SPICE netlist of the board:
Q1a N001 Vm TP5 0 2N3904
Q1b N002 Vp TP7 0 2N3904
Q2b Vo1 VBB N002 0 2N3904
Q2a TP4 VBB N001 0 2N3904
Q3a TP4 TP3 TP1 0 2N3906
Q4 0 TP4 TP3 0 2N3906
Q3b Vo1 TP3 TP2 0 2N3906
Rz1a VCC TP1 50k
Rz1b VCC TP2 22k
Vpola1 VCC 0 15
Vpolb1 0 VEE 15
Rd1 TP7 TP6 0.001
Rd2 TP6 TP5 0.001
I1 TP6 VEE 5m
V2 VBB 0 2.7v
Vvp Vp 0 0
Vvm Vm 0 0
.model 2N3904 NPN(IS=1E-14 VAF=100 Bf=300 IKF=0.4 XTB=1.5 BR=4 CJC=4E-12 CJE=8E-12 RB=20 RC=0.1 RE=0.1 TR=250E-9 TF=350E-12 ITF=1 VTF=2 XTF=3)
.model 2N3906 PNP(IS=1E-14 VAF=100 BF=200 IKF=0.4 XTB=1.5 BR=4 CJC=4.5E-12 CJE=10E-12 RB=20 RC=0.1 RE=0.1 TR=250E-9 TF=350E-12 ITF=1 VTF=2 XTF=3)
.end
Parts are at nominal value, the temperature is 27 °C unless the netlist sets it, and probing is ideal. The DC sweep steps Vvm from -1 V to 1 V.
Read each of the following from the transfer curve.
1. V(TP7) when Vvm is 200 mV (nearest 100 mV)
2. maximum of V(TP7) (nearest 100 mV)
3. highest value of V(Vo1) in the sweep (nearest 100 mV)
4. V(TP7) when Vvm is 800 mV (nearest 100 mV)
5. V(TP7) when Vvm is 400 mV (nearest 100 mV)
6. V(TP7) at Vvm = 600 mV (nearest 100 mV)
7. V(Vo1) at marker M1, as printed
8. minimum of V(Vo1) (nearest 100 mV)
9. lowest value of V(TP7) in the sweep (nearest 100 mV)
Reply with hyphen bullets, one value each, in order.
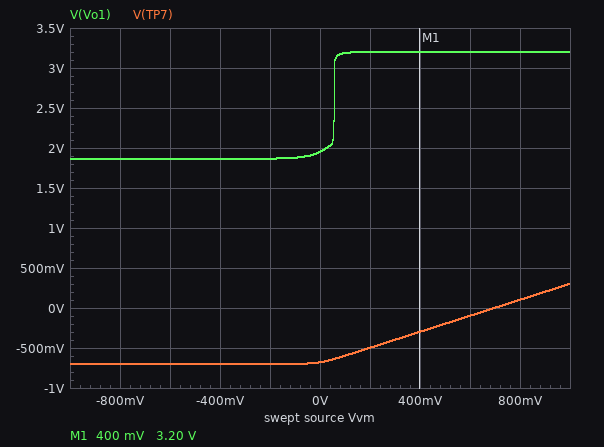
- -500 mV
- 300 mV
- 3.2 V
- 100 mV
- -300 mV
- -100 mV
- 3.20 V
- 1.9 V
- -700 mV
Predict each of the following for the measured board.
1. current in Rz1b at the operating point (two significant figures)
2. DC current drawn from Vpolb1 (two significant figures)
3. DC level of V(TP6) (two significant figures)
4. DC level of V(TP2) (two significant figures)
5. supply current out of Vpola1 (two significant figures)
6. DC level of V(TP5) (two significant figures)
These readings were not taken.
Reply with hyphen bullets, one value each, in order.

- 540 µA
- 5.0 mA
- -680 mV
- 3.1 V
- 780 µA
- -680 mV
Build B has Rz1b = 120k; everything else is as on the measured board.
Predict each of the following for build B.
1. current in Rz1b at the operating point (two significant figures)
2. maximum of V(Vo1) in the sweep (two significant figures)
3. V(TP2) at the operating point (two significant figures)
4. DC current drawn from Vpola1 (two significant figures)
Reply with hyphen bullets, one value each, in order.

- 100 µA
- 3.1 V
- 3.0 V
- 340 µA
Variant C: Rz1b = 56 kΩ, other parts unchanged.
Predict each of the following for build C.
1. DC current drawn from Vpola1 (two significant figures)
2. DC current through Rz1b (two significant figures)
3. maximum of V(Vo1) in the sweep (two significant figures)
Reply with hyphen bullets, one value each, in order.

- 450 µA
- 210 µA
- 3.1 V
